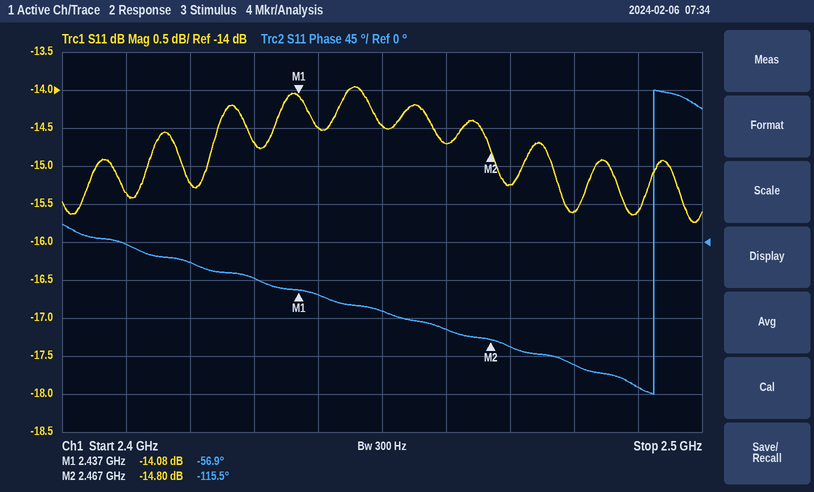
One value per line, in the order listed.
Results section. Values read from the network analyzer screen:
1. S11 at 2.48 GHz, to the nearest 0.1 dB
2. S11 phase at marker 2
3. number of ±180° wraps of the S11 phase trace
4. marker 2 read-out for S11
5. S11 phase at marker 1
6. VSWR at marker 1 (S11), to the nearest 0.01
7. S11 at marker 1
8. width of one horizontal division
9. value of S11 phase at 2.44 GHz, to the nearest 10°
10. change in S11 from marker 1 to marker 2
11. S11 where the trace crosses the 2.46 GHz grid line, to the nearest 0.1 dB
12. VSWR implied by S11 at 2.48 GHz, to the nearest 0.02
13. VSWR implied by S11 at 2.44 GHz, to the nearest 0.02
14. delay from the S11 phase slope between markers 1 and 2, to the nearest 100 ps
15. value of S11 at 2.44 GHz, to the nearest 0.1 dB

-15.6 dB
-115.5°
1
-14.80 dB
-56.9°
1.49
-14.08 dB
10 MHz
-60°
-0.72 dB
-14.7 dB
1.40
1.46
5.4 ns
-14.5 dB
